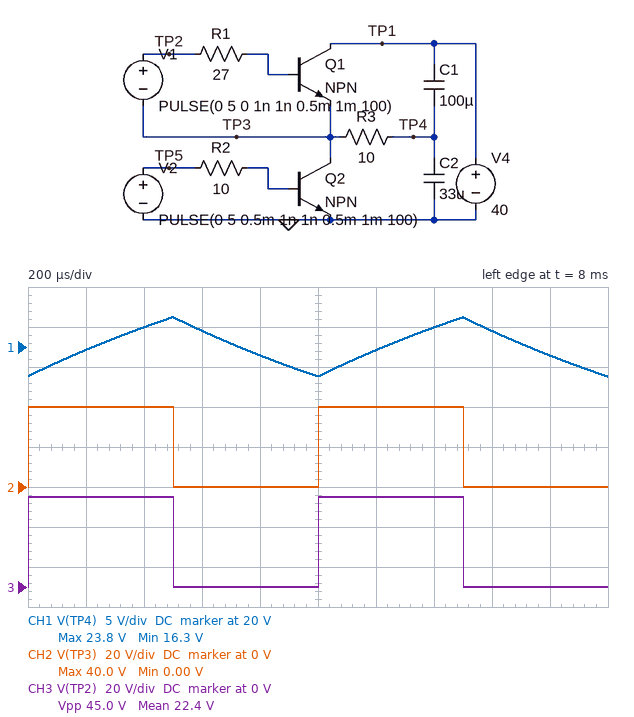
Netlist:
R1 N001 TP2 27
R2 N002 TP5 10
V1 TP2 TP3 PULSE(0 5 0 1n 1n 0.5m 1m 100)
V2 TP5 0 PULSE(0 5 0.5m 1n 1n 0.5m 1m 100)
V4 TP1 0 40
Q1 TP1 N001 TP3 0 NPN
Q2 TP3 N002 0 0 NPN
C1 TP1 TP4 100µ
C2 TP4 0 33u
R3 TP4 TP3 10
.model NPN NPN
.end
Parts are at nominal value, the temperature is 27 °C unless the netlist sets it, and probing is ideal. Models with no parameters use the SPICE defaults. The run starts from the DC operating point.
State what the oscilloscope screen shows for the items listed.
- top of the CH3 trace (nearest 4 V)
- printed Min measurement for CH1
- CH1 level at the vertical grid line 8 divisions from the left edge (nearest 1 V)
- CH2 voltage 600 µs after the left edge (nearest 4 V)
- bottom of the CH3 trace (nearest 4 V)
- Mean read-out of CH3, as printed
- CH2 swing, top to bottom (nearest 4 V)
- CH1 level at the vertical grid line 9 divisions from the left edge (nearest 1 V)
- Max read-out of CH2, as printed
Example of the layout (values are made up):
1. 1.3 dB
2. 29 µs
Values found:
1. 44 V
2. 16.3 V
3. 22 V
4. 0 V
5. 0 V
6. 22.4 V
7. 40 V
8. 19 V
9. 40.0 V
